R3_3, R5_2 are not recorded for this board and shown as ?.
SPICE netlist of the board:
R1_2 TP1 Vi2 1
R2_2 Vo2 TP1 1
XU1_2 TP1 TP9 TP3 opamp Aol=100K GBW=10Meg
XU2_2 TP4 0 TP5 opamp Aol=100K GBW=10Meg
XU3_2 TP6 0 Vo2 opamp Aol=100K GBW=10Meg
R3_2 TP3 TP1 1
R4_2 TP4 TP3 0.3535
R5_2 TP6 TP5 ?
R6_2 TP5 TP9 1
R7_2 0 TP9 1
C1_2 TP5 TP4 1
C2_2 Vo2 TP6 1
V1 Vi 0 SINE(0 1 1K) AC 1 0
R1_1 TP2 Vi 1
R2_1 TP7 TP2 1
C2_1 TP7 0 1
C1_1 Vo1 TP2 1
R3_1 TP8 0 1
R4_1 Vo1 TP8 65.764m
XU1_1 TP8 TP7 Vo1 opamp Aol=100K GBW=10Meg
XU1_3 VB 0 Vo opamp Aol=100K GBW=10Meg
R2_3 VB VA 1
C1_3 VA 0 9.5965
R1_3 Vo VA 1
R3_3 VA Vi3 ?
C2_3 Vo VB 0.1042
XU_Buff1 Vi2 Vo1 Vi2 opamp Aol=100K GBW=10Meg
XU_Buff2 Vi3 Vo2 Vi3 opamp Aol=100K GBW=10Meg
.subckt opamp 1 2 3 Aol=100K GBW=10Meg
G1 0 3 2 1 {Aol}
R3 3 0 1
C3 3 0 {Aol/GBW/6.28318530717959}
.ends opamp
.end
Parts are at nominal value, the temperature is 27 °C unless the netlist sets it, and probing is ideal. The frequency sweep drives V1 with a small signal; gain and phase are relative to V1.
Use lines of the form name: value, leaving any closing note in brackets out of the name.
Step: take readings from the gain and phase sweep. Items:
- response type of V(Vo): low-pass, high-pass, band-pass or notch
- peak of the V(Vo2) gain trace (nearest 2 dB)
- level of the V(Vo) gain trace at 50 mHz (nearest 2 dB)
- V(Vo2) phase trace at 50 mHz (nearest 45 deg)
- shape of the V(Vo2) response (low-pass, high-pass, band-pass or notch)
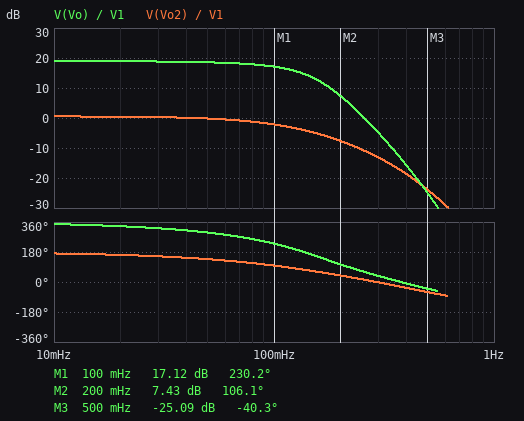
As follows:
response type of V(Vo): low-pass, high-pass, band-pass or notch: low-pass
peak of the V(Vo2) gain trace: 0 dB
level of the V(Vo) gain trace at 50 mHz: 18 dB
V(Vo2) phase trace at 50 mHz: 135 deg
shape of the V(Vo2) response: low-pass
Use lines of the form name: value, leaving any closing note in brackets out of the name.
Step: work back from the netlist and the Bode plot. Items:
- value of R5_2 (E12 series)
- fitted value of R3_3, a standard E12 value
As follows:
value of R5_2: 0.33 Ω
fitted value of R3_3, a standard E12 value: 0.12 Ω
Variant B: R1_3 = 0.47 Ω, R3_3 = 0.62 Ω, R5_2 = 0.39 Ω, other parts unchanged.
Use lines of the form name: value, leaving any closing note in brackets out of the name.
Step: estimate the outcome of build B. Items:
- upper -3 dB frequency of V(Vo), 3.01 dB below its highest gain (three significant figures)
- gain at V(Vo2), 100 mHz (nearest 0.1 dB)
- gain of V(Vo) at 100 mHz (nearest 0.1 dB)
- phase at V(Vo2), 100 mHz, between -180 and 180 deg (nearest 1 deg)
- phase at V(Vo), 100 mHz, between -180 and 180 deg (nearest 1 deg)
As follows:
upper -3 dB frequency of V(Vo), 3.01 dB below its highest gain: 246 mHz
gain at V(Vo2), 100 mHz: -2.2 dB
gain of V(Vo) at 100 mHz: -3.0 dB
phase at V(Vo2), 100 mHz, between -180 and 180 deg: 95 deg
phase at V(Vo), 100 mHz, between -180 and 180 deg: -95 deg
